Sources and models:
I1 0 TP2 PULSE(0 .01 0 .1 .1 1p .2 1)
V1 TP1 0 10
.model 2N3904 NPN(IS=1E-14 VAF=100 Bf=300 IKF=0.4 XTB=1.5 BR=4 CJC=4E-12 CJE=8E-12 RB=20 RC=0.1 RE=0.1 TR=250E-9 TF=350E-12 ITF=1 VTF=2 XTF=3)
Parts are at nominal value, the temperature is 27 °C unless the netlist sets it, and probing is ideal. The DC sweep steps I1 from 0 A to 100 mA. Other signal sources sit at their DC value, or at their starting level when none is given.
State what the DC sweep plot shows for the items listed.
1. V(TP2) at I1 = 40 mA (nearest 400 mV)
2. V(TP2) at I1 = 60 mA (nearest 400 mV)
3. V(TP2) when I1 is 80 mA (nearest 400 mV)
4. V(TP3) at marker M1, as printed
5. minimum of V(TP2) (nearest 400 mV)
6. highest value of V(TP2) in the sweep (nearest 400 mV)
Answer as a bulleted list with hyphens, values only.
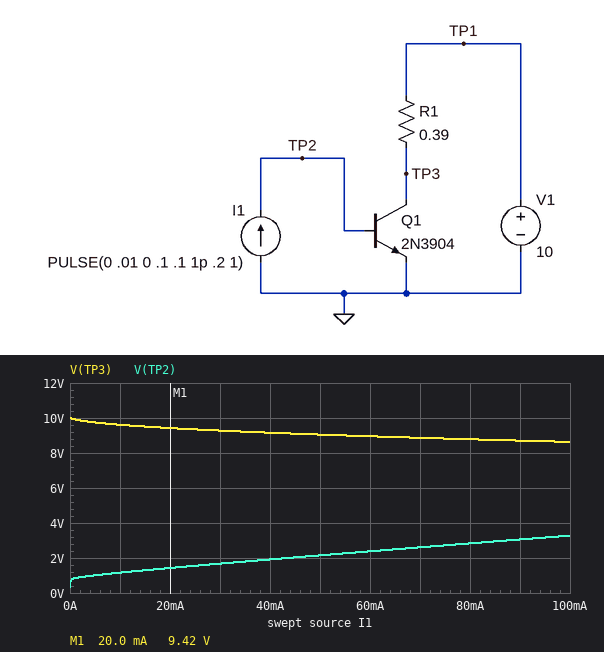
- 2.0 V
- 2.4 V
- 2.8 V
- 9.42 V
- 400 mV
- 3.2 V
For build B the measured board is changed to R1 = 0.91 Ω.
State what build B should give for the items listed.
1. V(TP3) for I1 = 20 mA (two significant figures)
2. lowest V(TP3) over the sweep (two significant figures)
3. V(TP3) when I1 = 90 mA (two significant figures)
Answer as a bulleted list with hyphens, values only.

- 8.7 V
- 6.9 V
- 7.0 V
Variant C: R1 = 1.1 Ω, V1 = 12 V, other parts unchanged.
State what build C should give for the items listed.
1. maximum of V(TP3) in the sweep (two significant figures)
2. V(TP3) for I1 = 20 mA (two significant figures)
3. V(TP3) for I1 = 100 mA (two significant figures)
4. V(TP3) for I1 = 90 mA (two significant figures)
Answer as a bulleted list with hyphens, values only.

- 12 V
- 10 V
- 8.2 V
- 8.4 V
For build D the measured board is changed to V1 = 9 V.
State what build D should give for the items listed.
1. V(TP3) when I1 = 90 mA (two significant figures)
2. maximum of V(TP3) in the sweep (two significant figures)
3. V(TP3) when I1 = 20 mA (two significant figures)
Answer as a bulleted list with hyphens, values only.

- 7.7 V
- 9.0 V
- 8.4 V
